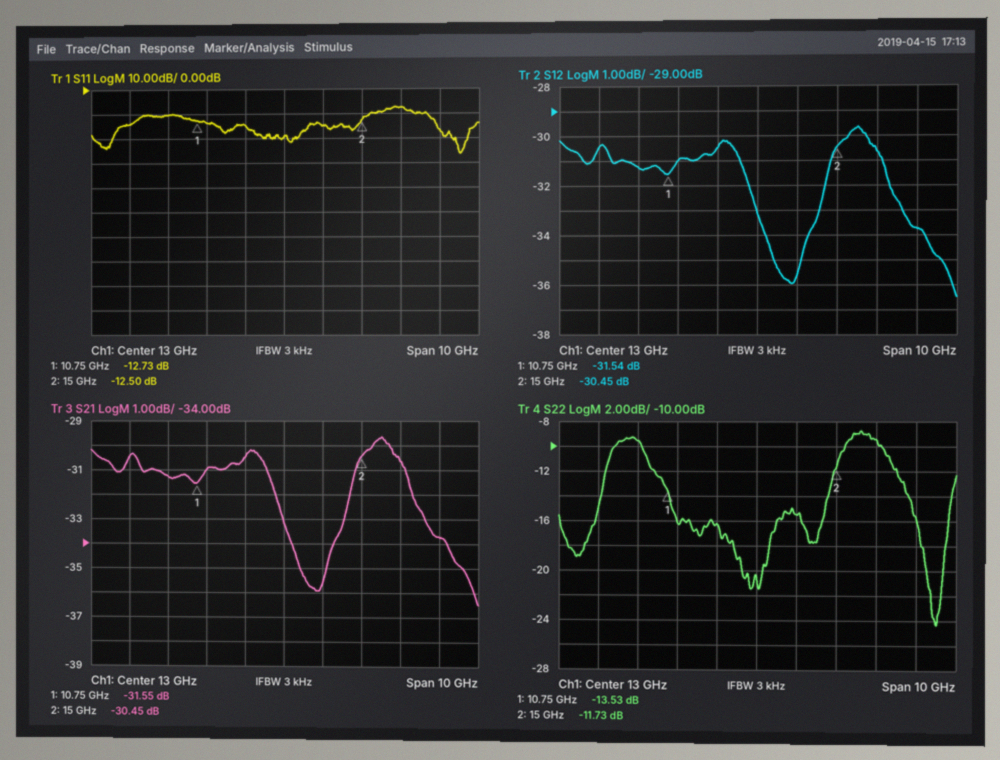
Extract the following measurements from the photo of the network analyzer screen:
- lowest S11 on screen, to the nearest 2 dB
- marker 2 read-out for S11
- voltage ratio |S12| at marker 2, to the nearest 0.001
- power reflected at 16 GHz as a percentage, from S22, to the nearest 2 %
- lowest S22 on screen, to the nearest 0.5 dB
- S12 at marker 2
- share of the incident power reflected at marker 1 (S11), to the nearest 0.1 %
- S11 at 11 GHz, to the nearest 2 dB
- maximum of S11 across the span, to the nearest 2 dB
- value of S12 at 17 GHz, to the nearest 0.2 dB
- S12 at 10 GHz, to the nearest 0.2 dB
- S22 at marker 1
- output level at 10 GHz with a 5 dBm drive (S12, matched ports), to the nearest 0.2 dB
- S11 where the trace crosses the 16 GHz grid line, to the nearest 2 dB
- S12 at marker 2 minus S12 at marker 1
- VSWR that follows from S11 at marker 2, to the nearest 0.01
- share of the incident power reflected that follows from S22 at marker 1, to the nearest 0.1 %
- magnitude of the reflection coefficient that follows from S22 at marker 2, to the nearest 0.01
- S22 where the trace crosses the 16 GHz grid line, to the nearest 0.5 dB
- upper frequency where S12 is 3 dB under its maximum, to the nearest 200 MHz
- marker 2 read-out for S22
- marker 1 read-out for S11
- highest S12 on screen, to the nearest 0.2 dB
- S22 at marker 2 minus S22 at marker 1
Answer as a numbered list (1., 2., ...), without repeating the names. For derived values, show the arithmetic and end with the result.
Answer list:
1. -26 dB
2. -12.50 dB
3. 10^(-30.45/20) ≈ 0.030
4. 10^(-9.5/10) ≈ 11.2 %, so 12 % to the nearest 2 %
5. -24.5 dB
6. -30.45 dB
7. 10^(-12.73/10) ≈ 5.3 %
8. -14 dB
9. -8 dB
10. -33.8 dB
11. -31.2 dB
12. -13.53 dB
13. 5 dBm + (-31.2 dB) = -26.2 dBm
14. -8 dB
15. -30.45 − (-31.54) = 1.09 dB
16. (1 + 0.2371)/(1 − 0.2371) ≈ 1.62
17. 10^(-13.53/10) ≈ 4.4 %
18. 10^(-11.73/20) ≈ 0.26
19. -9.5 dB
20. 16.6 GHz
21. -11.73 dB
22. -12.73 dB
23. -29.6 dB
24. -11.73 − (-13.53) = 1.80 dB
